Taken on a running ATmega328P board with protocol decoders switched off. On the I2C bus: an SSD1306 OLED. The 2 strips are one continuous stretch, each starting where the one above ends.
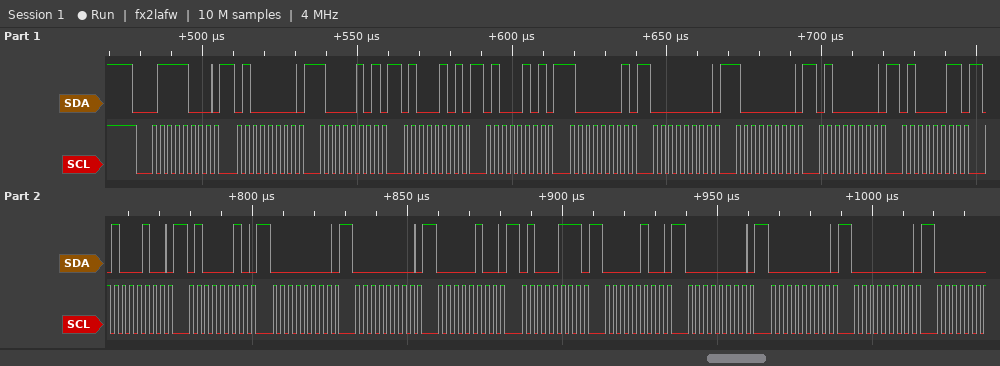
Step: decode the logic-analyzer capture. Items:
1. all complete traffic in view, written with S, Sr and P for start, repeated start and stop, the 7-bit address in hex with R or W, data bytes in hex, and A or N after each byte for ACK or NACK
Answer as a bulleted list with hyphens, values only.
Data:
- S 3CW A 40 A 85 A 45 A 45 A 81 A 00 A 80 A 40 A 43 A 44 A 42 A 00 A 00 A 04 A 47 A 04 A 00 A 00 A 00 A
